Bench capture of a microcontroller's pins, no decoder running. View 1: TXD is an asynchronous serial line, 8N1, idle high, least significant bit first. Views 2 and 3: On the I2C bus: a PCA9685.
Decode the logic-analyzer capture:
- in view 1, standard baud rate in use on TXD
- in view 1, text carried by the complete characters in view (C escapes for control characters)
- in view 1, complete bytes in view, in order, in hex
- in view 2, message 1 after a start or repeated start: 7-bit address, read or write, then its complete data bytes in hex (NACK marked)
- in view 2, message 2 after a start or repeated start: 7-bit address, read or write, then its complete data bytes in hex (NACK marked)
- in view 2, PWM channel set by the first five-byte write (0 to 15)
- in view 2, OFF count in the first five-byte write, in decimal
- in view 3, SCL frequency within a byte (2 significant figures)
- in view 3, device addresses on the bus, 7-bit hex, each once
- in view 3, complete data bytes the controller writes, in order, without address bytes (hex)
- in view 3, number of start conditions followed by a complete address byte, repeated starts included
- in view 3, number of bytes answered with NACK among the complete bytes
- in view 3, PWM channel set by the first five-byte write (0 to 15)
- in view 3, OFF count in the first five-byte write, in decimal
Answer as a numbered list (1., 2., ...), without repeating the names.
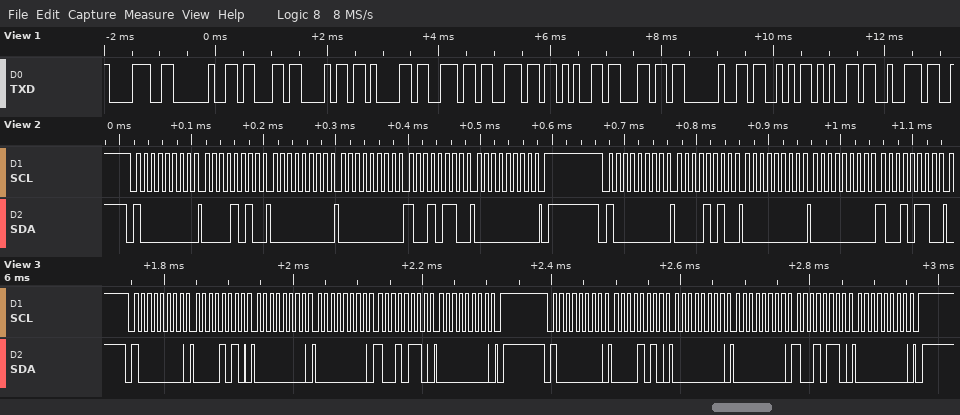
1. 9600 baud
2. "8 channel Ser"
3. 38 20 63 68 61 6E 6E 65 6C 20 53 65 72
4. 0x40 write: 0A 00 00 96 00
5. 0x40 write: 0A 00 00 96
6. 1
7. 150
8. 100 kHz
9. 0x40
10. 0A 00 00 96 00 0A 00 00 96 00
11. 2
12. 0
13. 1
14. 150
